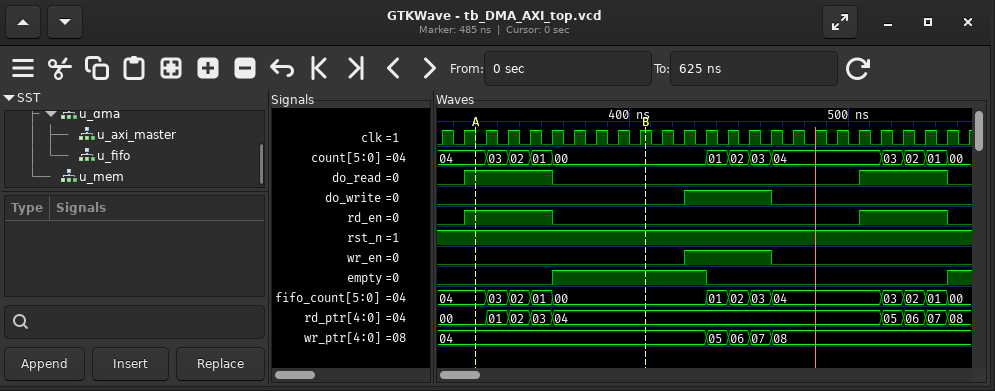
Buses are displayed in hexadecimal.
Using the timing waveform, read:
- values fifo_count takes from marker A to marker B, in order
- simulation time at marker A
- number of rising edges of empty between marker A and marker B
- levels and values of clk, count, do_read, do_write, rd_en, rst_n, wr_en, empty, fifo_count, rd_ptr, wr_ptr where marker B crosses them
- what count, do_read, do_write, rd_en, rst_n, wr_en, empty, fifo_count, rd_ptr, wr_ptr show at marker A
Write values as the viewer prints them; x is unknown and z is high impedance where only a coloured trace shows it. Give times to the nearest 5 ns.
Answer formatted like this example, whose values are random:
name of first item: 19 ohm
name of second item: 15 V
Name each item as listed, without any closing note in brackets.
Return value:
values fifo_count takes from marker A to marker B, in order: 04, 03, 02, 01, 00
simulation time at marker A: 330 ns
number of rising edges of empty between marker A and marker B: 1
levels and values of clk, count, do_read, do_write, rd_en, rst_n, wr_en, empty, fifo_count, rd_ptr, wr_ptr where marker B crosses them: clk=1, count=00, do_read=0, do_write=0, rd_en=0, rst_n=1, wr_en=0, empty=1, fifo_count=00, rd_ptr=04, wr_ptr=04
what count, do_read, do_write, rd_en, rst_n, wr_en, empty, fifo_count, rd_ptr, wr_ptr show at marker A: count=04, do_read=1, do_write=0, rd_en=1, rst_n=1, wr_en=0, empty=0, fifo_count=04, rd_ptr=00, wr_ptr=04
